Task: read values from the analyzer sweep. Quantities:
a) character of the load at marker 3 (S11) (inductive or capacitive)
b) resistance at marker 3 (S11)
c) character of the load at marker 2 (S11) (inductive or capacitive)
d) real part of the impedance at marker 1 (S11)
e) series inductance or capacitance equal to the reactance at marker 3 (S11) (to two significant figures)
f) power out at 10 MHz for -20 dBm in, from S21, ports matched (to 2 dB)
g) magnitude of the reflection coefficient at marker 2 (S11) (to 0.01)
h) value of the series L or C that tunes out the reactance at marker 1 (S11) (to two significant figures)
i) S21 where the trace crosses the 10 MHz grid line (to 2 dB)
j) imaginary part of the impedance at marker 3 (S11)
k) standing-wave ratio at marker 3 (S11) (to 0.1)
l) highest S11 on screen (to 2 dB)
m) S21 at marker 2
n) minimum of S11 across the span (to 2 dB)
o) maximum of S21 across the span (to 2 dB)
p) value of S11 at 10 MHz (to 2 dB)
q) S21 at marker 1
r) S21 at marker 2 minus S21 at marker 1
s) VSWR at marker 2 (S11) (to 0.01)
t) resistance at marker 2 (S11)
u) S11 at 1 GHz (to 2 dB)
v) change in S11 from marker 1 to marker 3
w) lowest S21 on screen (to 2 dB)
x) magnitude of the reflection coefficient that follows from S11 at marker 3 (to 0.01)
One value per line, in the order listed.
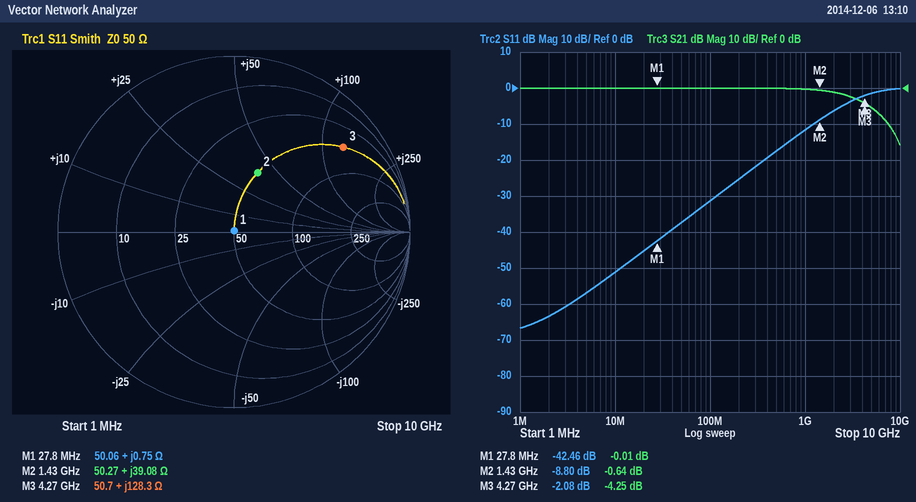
inductive
50.7 Ω
inductive
50.06 Ω
4.8 nH
-20 dBm
0.36
7.6 nF
0 dB
+128.3 Ω
8.4
0 dB
-0.64 dB
-66 dB
0 dB
-52 dB
-0.01 dB
-0.63 dB
2.14
50.27 Ω
-12 dB
40.38 dB
-16 dB
0.79
